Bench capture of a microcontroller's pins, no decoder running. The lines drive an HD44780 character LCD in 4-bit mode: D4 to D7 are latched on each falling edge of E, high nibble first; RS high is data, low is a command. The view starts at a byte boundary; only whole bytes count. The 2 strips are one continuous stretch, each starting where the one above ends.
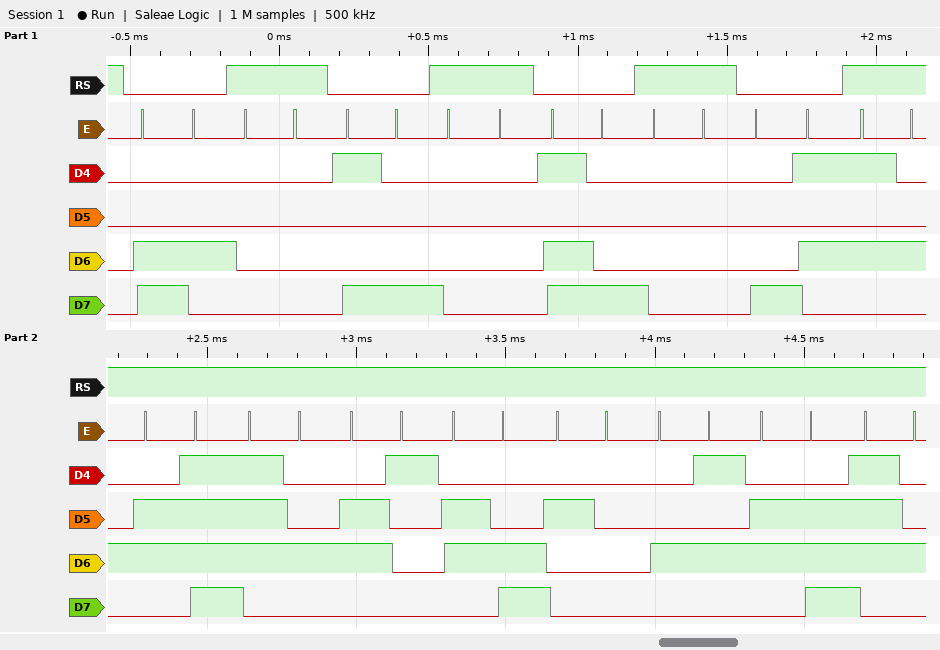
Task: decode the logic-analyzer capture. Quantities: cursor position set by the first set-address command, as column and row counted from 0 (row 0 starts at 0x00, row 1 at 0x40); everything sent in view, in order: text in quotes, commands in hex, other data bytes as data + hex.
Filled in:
column 4, row 1
0xC4 data 00 0x98 data 00 0xD8 data 00 0x85 "Total Ent"
